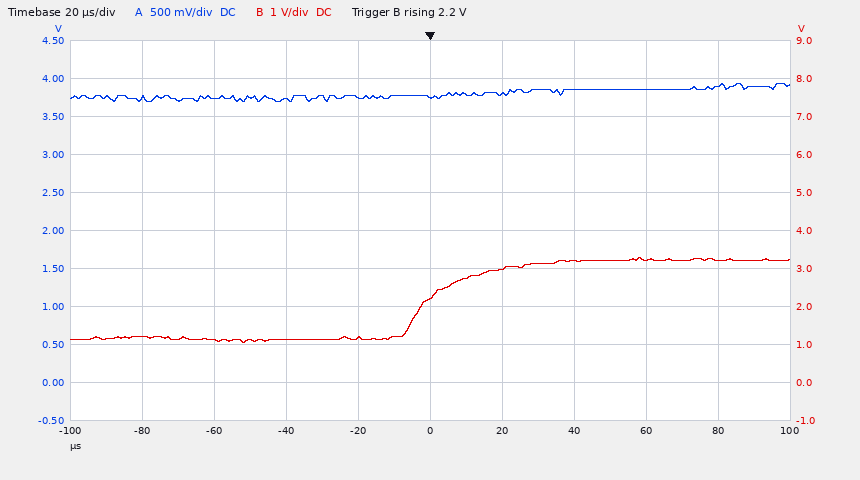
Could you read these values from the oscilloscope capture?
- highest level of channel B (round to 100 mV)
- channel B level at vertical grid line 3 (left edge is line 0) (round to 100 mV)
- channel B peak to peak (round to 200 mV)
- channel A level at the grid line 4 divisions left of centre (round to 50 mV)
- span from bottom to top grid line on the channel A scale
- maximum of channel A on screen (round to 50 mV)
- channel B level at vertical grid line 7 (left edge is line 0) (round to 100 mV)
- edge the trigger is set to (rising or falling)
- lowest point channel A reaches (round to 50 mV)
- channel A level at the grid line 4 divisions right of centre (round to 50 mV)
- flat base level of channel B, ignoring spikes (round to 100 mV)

3.3 V
1.1 V
2.2 V
3.75 V
5 V
3.95 V
3.2 V
rising
3.70 V
3.90 V
1.1 V
